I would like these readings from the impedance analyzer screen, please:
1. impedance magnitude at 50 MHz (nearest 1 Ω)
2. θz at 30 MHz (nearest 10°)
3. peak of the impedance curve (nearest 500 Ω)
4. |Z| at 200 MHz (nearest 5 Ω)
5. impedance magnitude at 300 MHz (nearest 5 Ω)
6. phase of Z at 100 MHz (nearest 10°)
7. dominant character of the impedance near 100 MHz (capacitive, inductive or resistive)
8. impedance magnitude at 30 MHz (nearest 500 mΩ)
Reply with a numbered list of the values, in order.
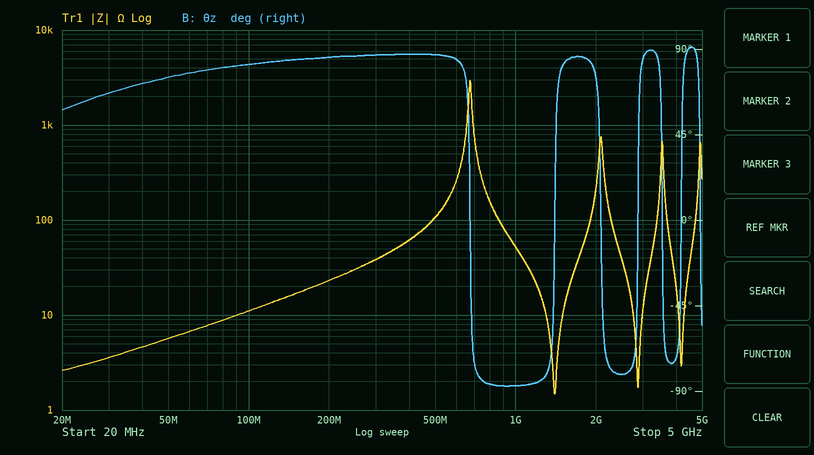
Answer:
1. 6 Ω
2. 70°
3. 3.0 kΩ
4. 25 Ω
5. 40 Ω
6. 80°
7. inductive
8. 3.5 Ω
